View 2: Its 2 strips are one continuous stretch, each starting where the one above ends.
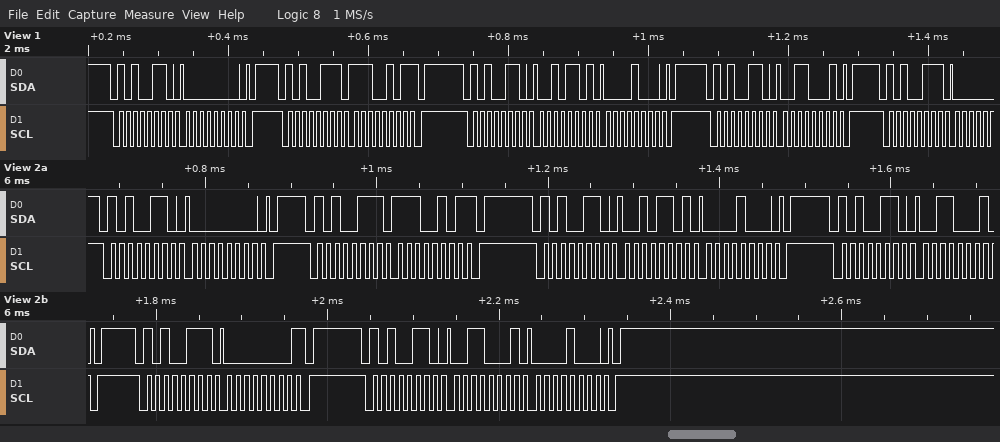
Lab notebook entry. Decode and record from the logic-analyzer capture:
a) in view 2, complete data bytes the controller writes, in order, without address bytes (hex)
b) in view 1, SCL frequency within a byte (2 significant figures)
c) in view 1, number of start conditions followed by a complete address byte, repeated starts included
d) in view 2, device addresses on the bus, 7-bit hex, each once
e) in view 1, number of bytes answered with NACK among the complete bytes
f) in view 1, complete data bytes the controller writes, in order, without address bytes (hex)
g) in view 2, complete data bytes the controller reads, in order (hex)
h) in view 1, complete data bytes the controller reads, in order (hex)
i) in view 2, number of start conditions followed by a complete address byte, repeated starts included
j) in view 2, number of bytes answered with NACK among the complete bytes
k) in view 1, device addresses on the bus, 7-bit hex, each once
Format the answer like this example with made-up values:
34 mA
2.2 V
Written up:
00 2D 08 31 31 08
100 kHz
5
0x53
1
00 2D 08 31
E5 00
E5
6
2
0x53
